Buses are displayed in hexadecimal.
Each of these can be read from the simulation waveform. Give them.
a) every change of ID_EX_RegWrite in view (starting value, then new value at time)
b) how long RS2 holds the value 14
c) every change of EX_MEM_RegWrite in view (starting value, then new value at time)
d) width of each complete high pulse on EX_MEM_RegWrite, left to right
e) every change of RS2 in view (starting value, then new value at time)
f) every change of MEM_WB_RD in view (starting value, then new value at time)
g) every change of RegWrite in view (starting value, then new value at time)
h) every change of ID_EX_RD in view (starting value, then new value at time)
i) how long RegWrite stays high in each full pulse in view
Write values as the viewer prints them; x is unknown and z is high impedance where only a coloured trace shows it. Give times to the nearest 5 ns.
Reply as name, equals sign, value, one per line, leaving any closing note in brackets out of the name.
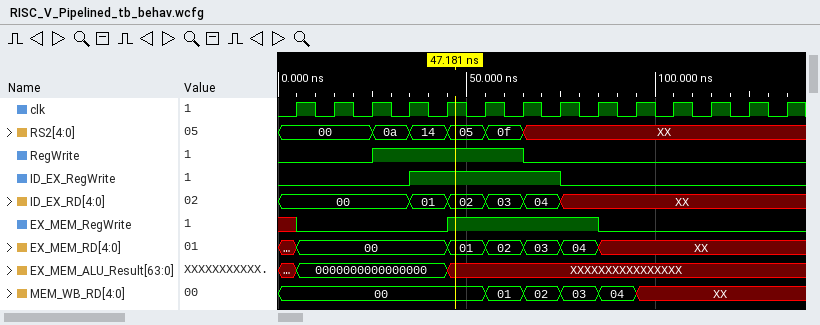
every change of ID_EX_RegWrite in view = 0, 1 at 35 ns, 0 at 75 ns
how long RS2 holds the value 14 = 10 ns
every change of EX_MEM_RegWrite in view = x, 0 at 5 ns, 1 at 45 ns, 0 at 85 ns
width of each complete high pulse on EX_MEM_RegWrite, left to right = 40 ns
every change of RS2 in view = 00, 0a at 25 ns, 14 at 35 ns, 05 at 45 ns, 0f at 55 ns, XX at 65 ns
every change of MEM_WB_RD in view = 00, 01 at 55 ns, 02 at 65 ns, 03 at 75 ns, 04 at 85 ns, XX at 95 ns
every change of RegWrite in view = 0, 1 at 25 ns, 0 at 65 ns
every change of ID_EX_RD in view = 00, 01 at 35 ns, 02 at 45 ns, 03 at 55 ns, 04 at 65 ns, XX at 75 ns
how long RegWrite stays high in each full pulse in view = 40 ns
